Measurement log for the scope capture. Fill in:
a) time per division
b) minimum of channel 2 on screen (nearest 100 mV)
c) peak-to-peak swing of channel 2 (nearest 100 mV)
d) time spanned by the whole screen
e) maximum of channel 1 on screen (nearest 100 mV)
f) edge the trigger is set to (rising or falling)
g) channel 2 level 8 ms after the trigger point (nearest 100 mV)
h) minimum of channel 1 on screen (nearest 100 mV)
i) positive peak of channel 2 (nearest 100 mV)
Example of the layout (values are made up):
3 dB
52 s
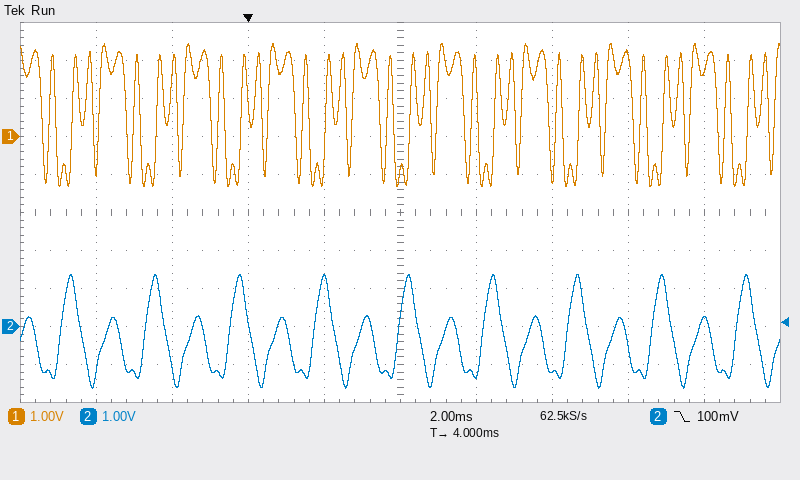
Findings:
2 ms
-1.6 V
3.0 V
20 ms
2.4 V
falling
-1.2 V
-1.3 V
1.4 V
